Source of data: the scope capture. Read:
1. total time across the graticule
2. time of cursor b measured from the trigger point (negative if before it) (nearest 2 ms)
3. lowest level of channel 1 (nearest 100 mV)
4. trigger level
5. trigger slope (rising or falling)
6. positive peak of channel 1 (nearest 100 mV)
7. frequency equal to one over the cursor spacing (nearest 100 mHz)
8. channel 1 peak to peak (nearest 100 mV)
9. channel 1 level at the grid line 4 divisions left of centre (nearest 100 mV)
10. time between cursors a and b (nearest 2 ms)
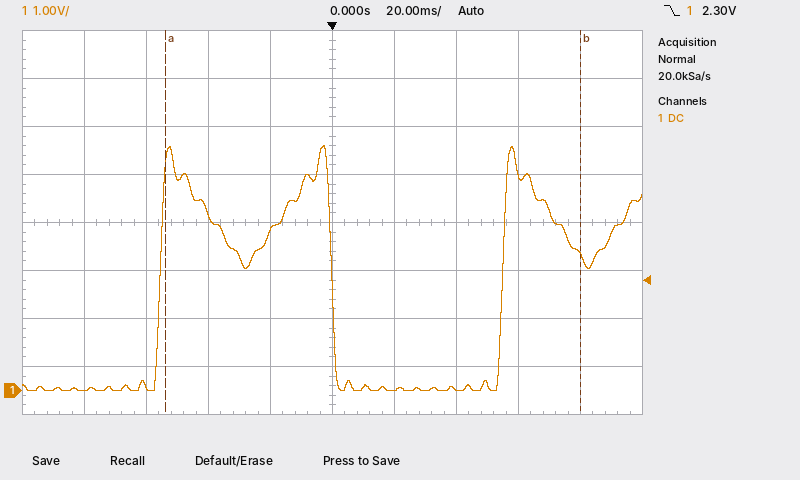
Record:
200 ms
+80 ms
0.0 V
2.30 V
falling
5.1 V
7.5 Hz
5.1 V
0.0 V
134 ms
